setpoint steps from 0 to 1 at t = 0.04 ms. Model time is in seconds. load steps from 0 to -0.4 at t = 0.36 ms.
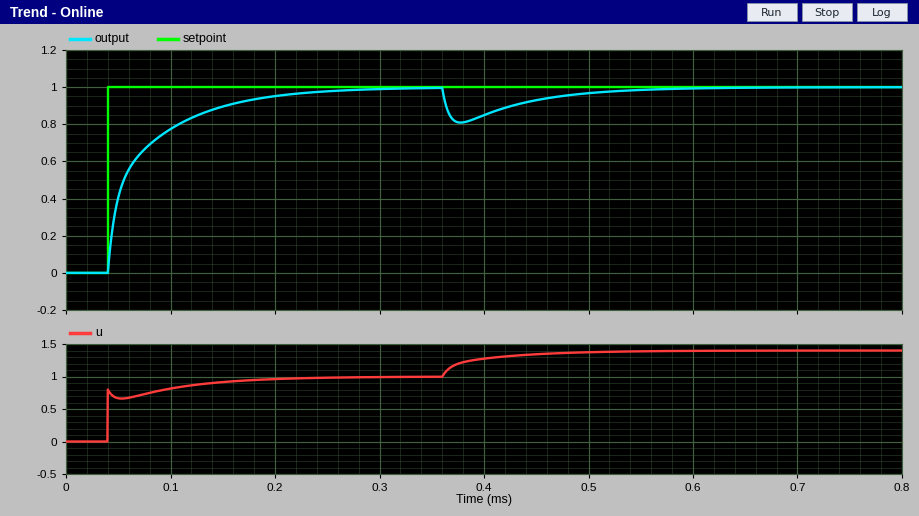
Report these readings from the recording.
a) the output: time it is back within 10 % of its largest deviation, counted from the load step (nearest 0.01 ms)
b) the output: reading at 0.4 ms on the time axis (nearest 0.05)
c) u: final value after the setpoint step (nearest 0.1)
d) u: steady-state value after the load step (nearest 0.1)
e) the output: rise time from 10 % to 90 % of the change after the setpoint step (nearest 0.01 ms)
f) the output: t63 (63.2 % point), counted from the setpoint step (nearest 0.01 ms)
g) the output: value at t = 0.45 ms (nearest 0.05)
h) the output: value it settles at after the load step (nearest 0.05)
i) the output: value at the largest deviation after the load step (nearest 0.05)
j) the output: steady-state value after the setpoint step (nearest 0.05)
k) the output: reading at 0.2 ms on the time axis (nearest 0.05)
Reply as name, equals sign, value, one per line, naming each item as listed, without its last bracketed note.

the output: time it is back within 10 % of its largest deviation, counted from the load step = 0.18 ms
the output: reading at 0.4 ms on the time axis = 0.85
u: final value after the setpoint step = 1.0
u: steady-state value after the load step = 1.4
the output: rise time from 10 % to 90 % of the change after the setpoint step = 0.11 ms
the output: t63 (63.2 % point), counted from the setpoint step = 0.03 ms
the output: value at t = 0.45 ms = 0.95
the output: value it settles at after the load step = 1.00
the output: value at the largest deviation after the load step = 0.80
the output: steady-state value after the setpoint step = 1.00
the output: reading at 0.2 ms on the time axis = 0.95
